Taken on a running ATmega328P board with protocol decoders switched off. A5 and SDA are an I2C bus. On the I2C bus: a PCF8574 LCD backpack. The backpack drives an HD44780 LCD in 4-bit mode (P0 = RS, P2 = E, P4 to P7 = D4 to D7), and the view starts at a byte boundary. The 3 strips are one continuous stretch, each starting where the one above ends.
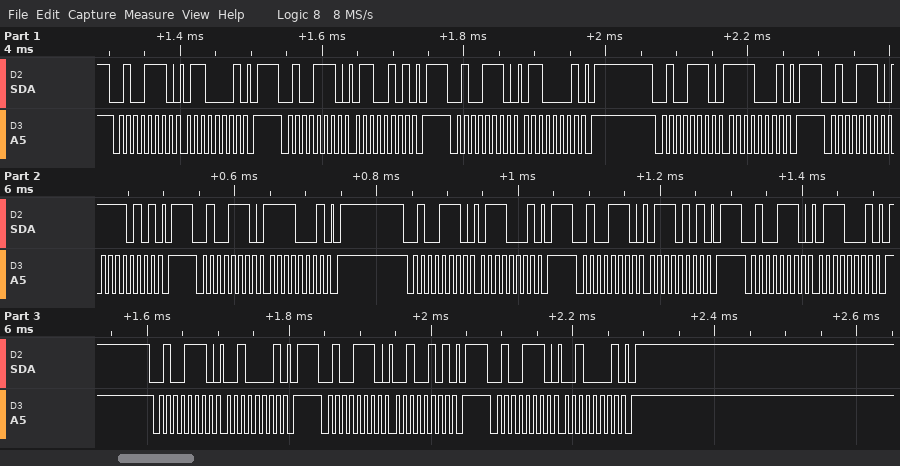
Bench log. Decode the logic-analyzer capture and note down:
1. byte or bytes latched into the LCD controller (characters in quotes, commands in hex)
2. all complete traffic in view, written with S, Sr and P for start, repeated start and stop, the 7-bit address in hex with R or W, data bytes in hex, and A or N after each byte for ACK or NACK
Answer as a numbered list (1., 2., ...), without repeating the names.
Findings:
1. 'o' 'r'
2. S 27W A 61 A P S 27W A 65 A P S 27W A 61 A P S 27W A F1 A P S 27W A F5 A P S 27W A F1 A P S 27W A 71 A P S 27W A 75 A P S 27W A 71 A P S 27W A 21 A P S 27W A 25 A P S 27W A 21 A P
